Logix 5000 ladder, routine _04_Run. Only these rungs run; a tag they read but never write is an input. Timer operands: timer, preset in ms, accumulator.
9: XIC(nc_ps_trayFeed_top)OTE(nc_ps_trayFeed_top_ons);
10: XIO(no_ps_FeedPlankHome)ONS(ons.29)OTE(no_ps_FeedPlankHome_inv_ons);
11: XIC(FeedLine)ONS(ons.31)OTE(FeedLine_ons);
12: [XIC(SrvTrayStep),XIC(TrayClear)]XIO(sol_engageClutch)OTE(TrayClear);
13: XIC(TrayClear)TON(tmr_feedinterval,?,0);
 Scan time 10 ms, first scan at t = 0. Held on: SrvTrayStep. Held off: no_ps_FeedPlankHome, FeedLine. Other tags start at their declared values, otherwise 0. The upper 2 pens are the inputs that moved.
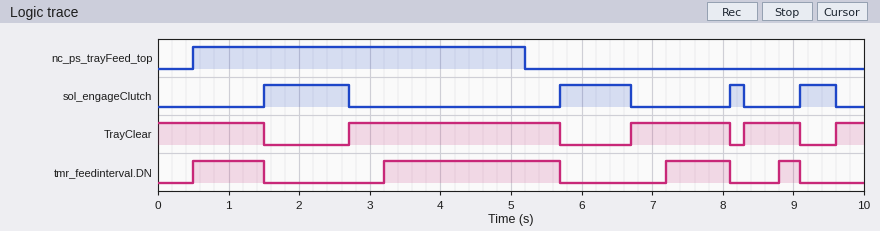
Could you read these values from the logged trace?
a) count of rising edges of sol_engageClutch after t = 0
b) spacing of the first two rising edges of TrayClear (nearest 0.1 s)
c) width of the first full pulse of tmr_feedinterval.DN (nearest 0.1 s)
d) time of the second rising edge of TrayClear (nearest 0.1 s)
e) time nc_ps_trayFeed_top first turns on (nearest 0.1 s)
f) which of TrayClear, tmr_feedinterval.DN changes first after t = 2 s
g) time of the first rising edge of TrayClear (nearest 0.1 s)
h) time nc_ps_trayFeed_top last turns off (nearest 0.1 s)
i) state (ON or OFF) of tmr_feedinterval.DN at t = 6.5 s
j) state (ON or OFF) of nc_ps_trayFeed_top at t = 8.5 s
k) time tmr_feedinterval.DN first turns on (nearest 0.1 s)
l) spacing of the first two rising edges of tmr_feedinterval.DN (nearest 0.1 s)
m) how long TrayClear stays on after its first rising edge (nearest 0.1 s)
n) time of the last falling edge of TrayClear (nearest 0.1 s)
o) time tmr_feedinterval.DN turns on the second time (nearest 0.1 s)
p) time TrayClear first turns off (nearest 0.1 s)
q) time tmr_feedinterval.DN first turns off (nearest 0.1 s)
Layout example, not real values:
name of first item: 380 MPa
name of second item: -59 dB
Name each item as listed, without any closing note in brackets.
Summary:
count of rising edges of sol_engageClutch after t = 0: 4
spacing of the first two rising edges of TrayClear: 4.0 s
width of the first full pulse of tmr_feedinterval.DN: 1.0 s
time of the second rising edge of TrayClear: 6.7 s
time nc_ps_trayFeed_top first turns on: 0.5 s
which of TrayClear, tmr_feedinterval.DN changes first after t = 2 s: TrayClear
time of the first rising edge of TrayClear: 2.7 s
time nc_ps_trayFeed_top last turns off: 5.2 s
state (ON or OFF) of tmr_feedinterval.DN at t = 6.5 s: OFF
state (ON or OFF) of nc_ps_trayFeed_top at t = 8.5 s: OFF
time tmr_feedinterval.DN first turns on: 0.5 s
spacing of the first two rising edges of tmr_feedinterval.DN: 2.7 s
how long TrayClear stays on after its first rising edge: 3.0 s
time of the last falling edge of TrayClear: 9.1 s
time tmr_feedinterval.DN turns on the second time: 3.2 s
time TrayClear first turns off: 1.5 s
time tmr_feedinterval.DN first turns off: 1.5 s
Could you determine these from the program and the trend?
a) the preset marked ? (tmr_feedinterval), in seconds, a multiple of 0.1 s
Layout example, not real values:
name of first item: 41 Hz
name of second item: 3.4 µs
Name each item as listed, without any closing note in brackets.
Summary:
the preset marked ? (tmr_feedinterval), in seconds, a multiple of 0.1 s: 0.5 s
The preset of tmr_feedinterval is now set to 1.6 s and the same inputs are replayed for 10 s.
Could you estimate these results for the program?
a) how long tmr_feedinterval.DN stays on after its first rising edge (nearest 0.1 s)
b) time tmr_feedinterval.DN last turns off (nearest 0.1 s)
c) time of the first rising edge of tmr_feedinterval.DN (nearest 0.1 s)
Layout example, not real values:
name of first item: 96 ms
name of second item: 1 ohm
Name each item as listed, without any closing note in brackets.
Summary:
how long tmr_feedinterval.DN stays on after its first rising edge: 1.4 s
time tmr_feedinterval.DN last turns off: 5.7 s
time of the first rising edge of tmr_feedinterval.DN: 4.3 s
